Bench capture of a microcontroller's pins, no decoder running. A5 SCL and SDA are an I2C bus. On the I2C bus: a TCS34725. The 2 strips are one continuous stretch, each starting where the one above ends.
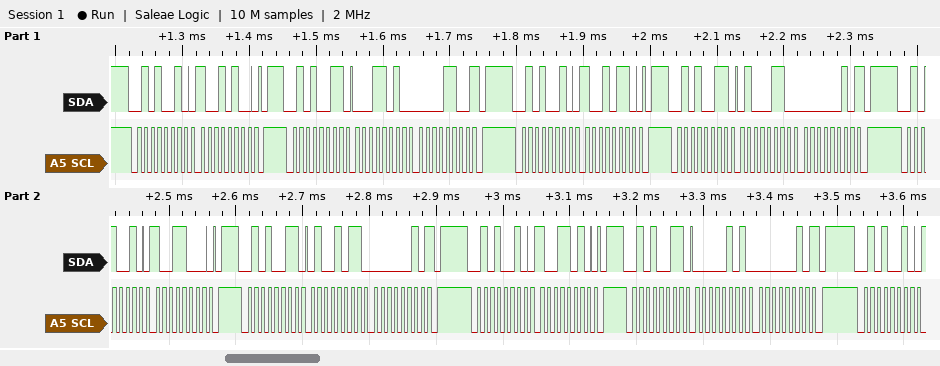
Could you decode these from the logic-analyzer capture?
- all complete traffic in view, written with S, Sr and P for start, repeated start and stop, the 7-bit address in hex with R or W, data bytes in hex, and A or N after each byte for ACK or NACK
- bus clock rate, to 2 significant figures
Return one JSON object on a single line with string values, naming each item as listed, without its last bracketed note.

{"all complete traffic in view, written with S, Sr and P for start, repeated start and stop, the 7-bit address in hex with R or W, data bytes in hex, and A or N after each byte for ACK or NACK": "S 29W A 94 A P S 29R A 1A A 0C N P S 29W A 96 A P S 29R A 46 A 02 N P S 29W A 98 A P S 29R A 4B A 02 N P S 29W A 9A A P S 29R A 05 A 02 N P S 29W A", "bus clock rate, to 2 significant figures": "100 kHz"}
